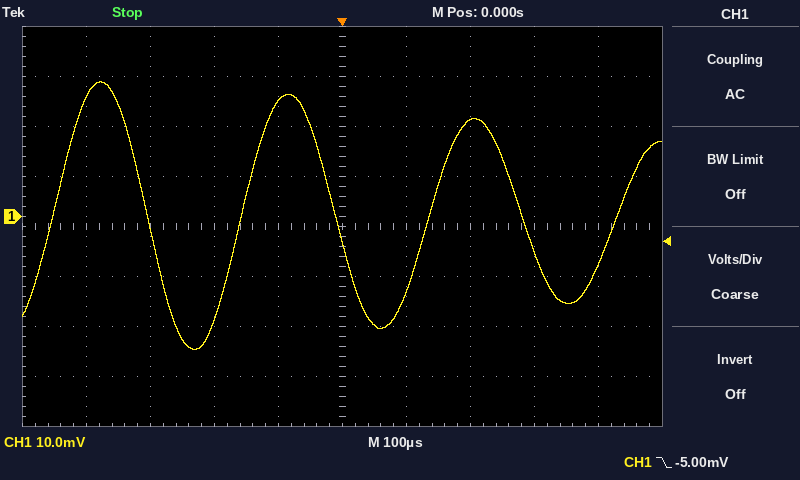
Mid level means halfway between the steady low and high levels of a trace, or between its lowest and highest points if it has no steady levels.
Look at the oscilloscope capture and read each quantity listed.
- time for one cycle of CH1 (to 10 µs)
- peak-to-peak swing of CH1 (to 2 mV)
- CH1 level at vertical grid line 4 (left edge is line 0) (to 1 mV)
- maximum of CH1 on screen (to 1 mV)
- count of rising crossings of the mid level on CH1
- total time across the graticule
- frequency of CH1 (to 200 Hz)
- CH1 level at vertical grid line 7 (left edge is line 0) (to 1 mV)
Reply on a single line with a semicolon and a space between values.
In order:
290 µs; 54 mV; 23 mV; 27 mV; 4; 1 ms; 3.4 kHz; 19 mV
